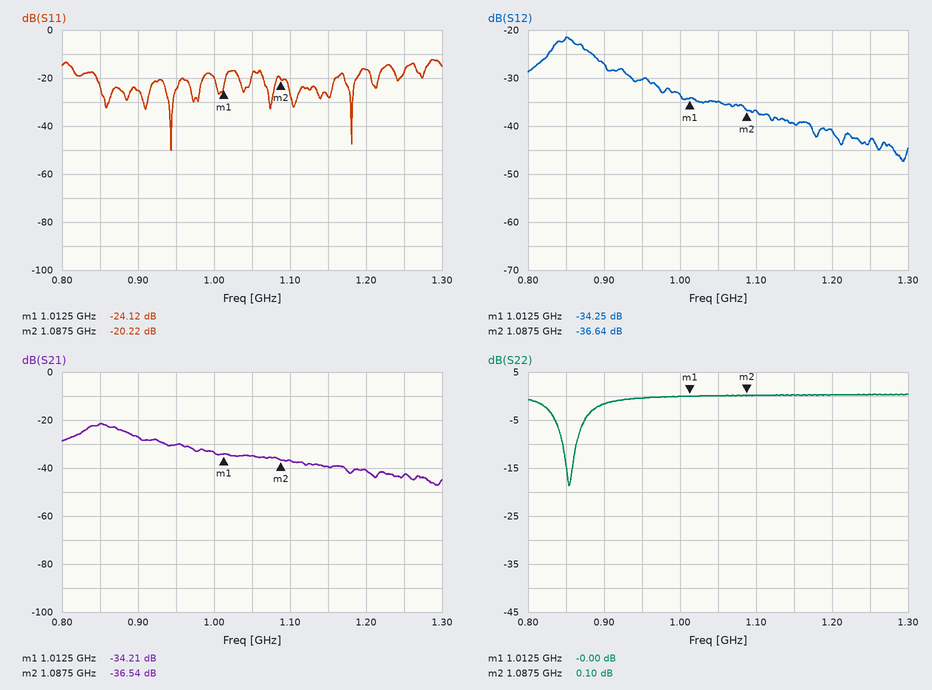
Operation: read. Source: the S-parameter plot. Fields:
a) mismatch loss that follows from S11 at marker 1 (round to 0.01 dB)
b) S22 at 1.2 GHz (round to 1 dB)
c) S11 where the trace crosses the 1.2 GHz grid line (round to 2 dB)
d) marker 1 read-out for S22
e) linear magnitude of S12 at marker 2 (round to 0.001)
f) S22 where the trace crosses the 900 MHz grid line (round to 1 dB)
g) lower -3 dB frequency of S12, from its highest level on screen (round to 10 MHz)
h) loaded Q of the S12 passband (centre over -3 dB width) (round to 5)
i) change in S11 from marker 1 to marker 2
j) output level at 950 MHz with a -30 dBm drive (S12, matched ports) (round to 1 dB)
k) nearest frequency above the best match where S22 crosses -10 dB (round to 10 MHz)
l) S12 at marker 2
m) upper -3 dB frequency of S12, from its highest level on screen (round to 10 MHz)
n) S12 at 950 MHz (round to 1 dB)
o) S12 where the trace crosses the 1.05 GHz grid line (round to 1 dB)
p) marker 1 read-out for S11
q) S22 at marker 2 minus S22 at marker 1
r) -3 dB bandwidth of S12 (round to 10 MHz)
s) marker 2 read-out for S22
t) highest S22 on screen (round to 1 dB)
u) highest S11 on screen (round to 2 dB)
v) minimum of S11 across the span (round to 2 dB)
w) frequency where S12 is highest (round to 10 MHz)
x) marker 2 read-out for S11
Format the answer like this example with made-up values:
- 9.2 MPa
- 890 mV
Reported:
- 0.02 dB
- 0 dB
- -16 dB
- -0.00 dB
- 0.015
- -2 dB
- 830 MHz
- 15
- 3.90 dB
- -60 dBm
- 860 MHz
- -36.64 dB
- 880 MHz
- -30 dB
- -35 dB
- -24.12 dB
- 0.10 dB
- 50 MHz
- 0.10 dB
- 0 dB
- -12 dB
- -50 dB
- 850 MHz
- -20.22 dB
